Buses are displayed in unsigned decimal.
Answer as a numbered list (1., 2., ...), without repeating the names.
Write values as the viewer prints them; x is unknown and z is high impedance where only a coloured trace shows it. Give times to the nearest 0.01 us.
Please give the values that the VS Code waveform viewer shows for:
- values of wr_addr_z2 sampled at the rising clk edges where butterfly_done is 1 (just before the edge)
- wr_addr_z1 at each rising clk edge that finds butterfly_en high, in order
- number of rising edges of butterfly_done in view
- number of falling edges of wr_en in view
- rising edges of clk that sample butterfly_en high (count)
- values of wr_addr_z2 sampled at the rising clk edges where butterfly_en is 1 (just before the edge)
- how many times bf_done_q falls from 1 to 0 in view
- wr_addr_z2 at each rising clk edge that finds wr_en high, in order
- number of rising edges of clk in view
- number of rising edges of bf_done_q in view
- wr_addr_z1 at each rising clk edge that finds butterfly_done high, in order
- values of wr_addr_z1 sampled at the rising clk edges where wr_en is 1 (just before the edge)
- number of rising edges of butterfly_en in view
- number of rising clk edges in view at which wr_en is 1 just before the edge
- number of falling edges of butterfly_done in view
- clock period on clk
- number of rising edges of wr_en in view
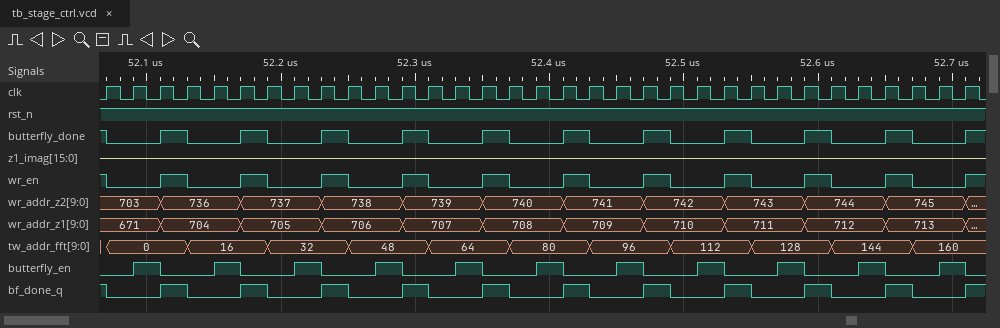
1. 703, 736, 737, 738, 739, 740, 741, 742, 743, 744, 745
2. 671, 704, 705, 706, 707, 708, 709, 710, 711, 712, 713
3. 11
4. 11
5. 11
6. 703, 736, 737, 738, 739, 740, 741, 742, 743, 744, 745
7. 11
8. 703, 736, 737, 738, 739, 740, 741, 742, 743, 744, 745
9. 33
10. 11
11. 671, 704, 705, 706, 707, 708, 709, 710, 711, 712, 713
12. 671, 704, 705, 706, 707, 708, 709, 710, 711, 712, 713
13. 11
14. 11
15. 11
16. 0.02 us
17. 11
